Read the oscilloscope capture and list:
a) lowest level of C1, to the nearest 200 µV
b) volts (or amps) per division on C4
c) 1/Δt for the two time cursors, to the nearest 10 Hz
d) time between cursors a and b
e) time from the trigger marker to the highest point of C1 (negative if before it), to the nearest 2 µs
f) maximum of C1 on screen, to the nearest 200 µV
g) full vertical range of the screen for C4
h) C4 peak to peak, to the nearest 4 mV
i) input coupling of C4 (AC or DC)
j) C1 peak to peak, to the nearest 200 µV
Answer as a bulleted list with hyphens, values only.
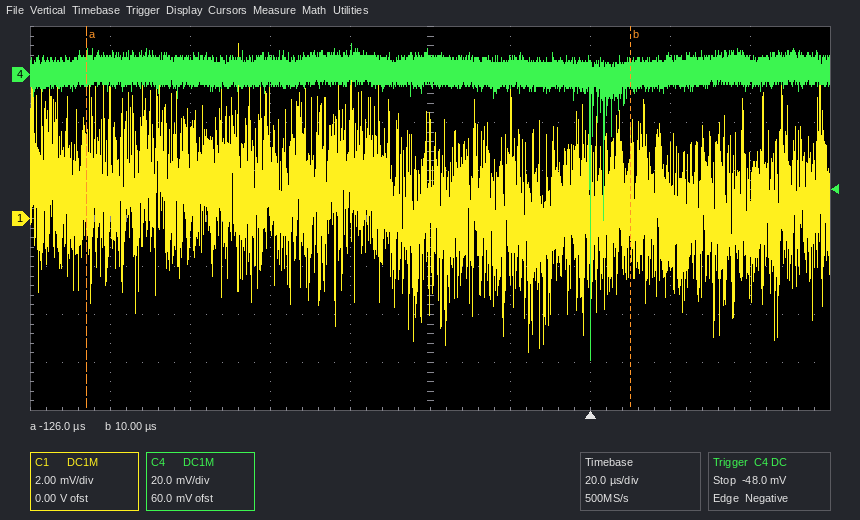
- -5.6 mV
- 20 mV
- 7.35 kHz
- 136 µs
- -88 µs
- 7.2 mV
- 160 mV
- 132 mV
- DC
- 12.8 mV
